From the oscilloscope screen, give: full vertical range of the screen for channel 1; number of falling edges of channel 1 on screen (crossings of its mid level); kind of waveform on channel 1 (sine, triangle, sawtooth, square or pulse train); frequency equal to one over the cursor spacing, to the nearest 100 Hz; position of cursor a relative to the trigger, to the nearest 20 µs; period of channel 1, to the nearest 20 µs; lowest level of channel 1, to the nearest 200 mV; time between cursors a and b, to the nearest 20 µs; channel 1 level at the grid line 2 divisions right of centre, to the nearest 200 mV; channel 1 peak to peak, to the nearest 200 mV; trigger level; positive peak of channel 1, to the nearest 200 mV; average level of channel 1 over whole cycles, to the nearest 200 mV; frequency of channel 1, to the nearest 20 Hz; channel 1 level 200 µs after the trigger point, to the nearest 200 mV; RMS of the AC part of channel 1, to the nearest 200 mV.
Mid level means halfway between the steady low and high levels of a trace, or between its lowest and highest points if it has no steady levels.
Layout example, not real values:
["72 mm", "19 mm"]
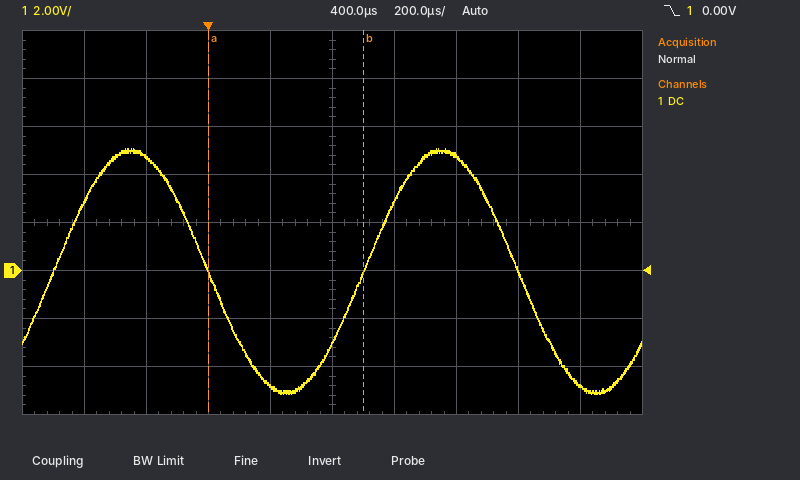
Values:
["16 V", "2", "sine", "2.0 kHz", "0 µs", "1.00 ms", "-5.2 V", "500 µs", "4.8 V", "10.2 V", "0.00 V", "5.0 V", "0.0 V", "1.00 kHz", "-4.8 V", "3.6 V"]
